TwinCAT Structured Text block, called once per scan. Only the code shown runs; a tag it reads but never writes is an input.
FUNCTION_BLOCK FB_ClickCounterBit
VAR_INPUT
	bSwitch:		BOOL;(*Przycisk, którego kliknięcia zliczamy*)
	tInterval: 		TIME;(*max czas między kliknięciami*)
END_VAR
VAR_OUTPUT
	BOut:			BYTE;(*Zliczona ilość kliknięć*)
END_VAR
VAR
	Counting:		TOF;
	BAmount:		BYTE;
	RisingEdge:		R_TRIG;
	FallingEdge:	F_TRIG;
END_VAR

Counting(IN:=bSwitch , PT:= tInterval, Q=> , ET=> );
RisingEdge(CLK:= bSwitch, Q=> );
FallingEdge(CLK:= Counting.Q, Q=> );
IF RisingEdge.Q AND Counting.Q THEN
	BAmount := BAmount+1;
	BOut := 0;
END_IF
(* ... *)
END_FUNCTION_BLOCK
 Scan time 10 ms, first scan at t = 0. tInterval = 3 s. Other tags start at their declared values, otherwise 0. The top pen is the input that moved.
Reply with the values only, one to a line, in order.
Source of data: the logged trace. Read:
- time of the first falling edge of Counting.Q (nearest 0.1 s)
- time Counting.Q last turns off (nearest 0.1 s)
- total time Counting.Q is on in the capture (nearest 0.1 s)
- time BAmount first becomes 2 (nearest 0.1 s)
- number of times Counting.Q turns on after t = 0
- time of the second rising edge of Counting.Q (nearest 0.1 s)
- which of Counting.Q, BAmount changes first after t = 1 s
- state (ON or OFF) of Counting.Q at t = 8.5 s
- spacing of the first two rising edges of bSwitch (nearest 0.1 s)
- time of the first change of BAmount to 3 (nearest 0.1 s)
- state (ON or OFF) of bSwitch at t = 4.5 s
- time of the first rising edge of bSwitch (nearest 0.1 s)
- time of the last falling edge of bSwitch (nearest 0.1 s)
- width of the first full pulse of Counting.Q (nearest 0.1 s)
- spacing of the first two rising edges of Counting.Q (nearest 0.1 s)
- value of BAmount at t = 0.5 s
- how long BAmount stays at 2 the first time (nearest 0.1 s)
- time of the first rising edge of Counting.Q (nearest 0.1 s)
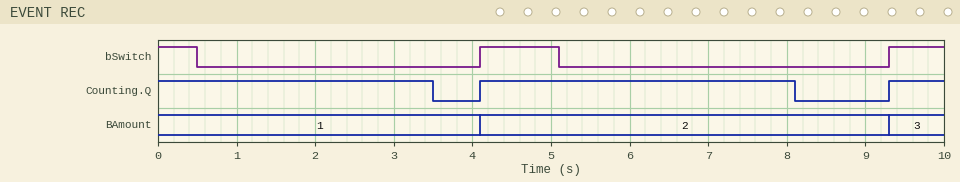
3.5 s
8.1 s
8.2 s
4.1 s
2
9.3 s
Counting.Q
OFF
5.2 s
9.3 s
ON
4.1 s
5.1 s
4.0 s
5.2 s
1
5.2 s
4.1 s
